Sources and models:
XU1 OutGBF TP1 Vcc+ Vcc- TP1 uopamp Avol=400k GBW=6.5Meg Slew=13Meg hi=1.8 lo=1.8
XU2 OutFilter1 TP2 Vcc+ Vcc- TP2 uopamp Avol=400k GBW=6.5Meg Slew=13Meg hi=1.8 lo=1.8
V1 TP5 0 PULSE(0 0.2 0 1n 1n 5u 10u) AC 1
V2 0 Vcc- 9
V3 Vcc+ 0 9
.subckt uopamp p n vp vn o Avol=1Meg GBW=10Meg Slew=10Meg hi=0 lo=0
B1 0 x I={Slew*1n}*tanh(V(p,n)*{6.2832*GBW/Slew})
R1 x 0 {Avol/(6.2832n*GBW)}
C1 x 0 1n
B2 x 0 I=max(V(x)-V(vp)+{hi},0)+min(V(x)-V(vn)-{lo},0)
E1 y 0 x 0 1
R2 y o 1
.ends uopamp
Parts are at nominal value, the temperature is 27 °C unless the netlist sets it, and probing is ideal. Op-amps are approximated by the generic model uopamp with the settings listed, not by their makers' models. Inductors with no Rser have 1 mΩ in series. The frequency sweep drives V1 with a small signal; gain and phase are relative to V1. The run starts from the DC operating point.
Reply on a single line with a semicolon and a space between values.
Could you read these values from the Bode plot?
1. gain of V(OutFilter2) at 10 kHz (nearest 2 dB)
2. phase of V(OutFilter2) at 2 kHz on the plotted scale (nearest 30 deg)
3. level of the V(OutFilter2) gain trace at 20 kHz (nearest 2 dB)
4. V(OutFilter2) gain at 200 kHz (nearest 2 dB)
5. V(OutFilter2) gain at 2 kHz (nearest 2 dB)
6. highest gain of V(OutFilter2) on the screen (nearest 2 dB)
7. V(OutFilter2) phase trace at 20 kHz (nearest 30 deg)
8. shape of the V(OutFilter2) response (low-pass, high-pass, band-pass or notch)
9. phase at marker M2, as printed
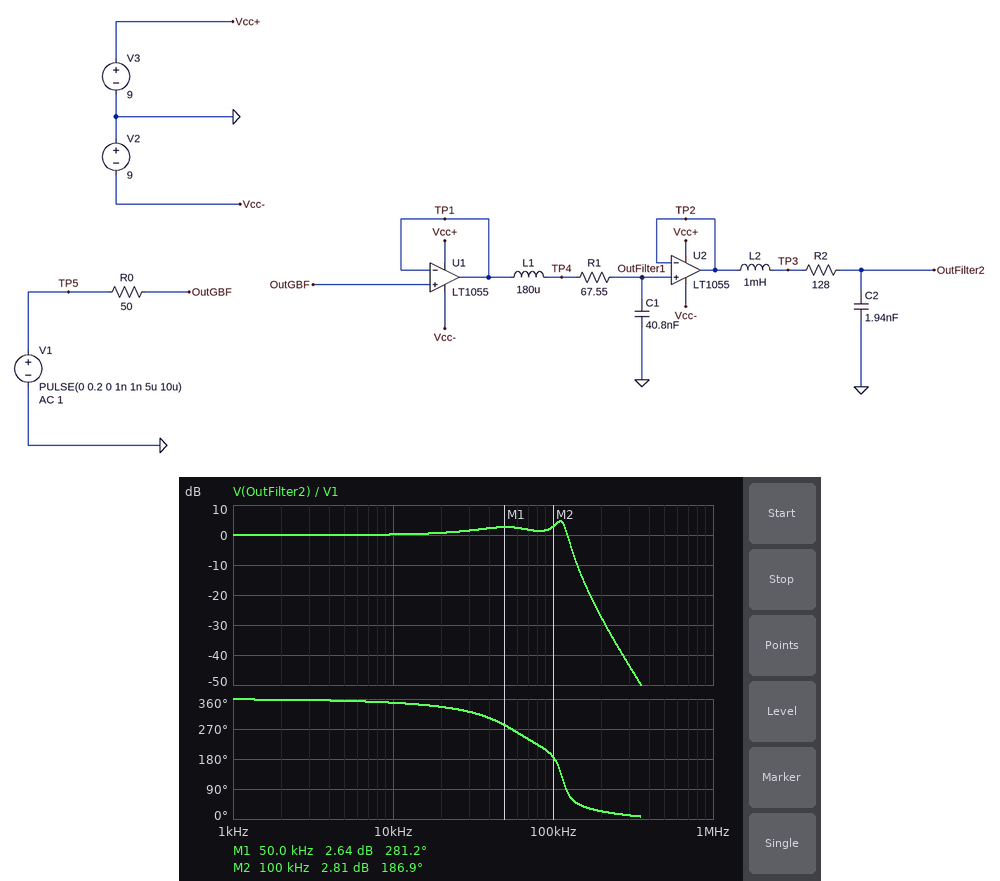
0 dB; 360 deg; 0 dB; -28 dB; 0 dB; 4 dB; 330 deg; low-pass; 186.9 deg
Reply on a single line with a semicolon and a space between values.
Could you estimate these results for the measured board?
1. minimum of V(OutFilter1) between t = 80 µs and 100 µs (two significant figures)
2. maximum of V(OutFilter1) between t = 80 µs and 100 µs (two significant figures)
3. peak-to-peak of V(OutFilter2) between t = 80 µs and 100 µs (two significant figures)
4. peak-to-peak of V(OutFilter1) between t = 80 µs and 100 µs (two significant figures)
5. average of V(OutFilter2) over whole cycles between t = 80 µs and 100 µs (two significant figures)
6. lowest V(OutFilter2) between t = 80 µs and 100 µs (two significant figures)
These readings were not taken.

50 mV; 150 mV; 350 mV; 100 mV; 100 mV; -76 mV
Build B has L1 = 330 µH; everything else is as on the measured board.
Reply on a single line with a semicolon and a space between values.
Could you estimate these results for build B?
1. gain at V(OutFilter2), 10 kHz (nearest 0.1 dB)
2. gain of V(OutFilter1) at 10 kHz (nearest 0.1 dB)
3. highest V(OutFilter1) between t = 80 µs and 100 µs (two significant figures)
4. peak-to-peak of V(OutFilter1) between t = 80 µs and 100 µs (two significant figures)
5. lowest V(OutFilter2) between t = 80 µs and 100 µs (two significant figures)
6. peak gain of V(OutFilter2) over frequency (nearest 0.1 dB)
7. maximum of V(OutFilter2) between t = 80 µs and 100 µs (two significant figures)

0.4 dB; 0.3 dB; 130 mV; 54 mV; 2.6 mV; 4.1 dB; 200 mV
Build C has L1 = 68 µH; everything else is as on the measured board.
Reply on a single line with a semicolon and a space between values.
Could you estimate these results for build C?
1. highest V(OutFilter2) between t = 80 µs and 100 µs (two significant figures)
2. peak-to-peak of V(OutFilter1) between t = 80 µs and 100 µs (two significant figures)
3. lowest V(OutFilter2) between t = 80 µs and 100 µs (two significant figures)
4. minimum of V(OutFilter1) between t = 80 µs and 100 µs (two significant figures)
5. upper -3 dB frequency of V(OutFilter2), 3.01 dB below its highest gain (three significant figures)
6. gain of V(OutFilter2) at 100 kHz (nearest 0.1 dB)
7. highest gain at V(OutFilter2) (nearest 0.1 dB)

360 mV; 160 mV; -160 mV; 22 mV; 121 kHz; 6.2 dB; 9.0 dB
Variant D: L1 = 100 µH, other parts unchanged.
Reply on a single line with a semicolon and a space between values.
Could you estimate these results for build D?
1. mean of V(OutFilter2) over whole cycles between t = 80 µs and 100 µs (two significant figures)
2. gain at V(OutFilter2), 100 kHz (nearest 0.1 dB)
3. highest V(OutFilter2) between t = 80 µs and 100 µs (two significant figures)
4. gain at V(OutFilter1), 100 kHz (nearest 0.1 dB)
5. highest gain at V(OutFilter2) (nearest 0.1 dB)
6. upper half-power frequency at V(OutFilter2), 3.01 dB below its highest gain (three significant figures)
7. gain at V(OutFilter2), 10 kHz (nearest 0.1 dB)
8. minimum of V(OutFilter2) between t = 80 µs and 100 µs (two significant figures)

100 mV; 5.7 dB; 350 mV; -5.3 dB; 8.1 dB; 121 kHz; 0.1 dB; -150 mV
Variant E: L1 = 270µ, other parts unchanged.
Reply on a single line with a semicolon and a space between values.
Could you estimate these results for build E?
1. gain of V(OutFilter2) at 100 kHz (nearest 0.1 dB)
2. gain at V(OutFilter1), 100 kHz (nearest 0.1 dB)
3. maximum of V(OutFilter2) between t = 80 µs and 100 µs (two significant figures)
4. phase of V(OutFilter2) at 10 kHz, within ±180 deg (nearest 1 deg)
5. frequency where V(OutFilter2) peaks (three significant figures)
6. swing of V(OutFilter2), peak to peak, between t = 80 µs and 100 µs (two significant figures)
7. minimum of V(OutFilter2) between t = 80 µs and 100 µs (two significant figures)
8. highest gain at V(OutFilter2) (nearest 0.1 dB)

-0.5 dB; -11.5 dB; 220 mV; -11 deg; 42.1 kHz; 240 mV; -20 mV; 3.6 dB
